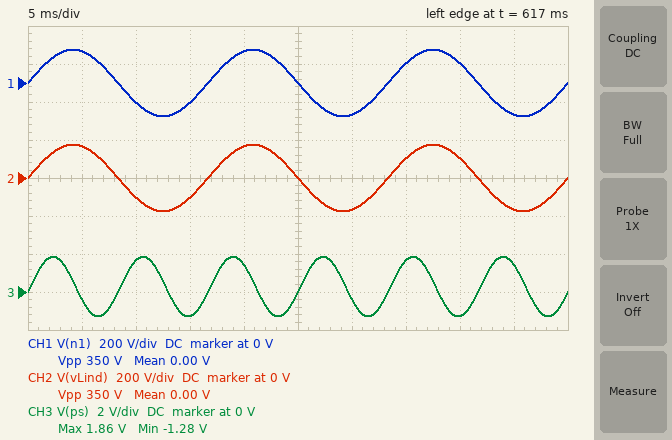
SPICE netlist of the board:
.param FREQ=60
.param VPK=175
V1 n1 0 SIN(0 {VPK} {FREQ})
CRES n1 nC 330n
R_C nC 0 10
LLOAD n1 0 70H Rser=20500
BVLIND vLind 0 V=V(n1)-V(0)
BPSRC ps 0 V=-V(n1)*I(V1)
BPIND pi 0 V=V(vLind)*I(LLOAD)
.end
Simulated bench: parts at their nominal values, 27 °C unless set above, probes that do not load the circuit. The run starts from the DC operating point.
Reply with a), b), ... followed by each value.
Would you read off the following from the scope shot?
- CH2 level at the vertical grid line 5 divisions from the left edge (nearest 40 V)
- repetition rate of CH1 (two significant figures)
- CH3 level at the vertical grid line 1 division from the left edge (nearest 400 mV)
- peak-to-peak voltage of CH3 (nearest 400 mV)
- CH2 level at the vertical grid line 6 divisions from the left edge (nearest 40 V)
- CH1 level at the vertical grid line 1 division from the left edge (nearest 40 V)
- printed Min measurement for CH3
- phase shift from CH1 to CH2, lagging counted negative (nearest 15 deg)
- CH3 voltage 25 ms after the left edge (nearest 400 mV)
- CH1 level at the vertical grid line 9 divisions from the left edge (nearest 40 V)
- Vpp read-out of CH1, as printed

a) 0 V
b) 60 Hz
c) -400 mV
d) 3.2 V
e) -160 V
f) 160 V
g) -1.28 V
h) 0 deg
i) 0 V
j) -160 V
k) 350 V
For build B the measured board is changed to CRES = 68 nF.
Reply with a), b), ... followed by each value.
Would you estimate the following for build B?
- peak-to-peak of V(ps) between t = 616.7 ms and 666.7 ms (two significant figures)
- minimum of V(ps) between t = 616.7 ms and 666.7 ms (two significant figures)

a) 570 mV
b) -1.7 mV
